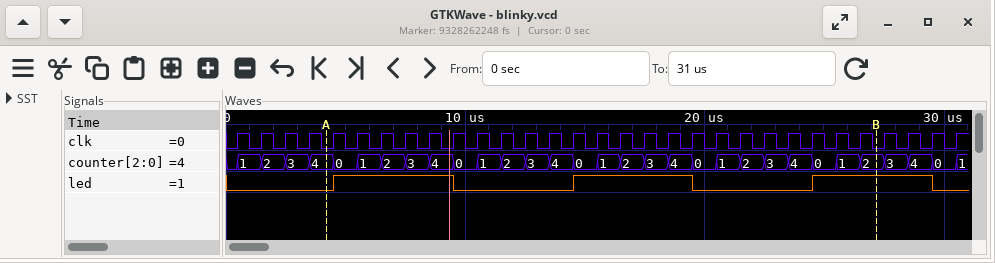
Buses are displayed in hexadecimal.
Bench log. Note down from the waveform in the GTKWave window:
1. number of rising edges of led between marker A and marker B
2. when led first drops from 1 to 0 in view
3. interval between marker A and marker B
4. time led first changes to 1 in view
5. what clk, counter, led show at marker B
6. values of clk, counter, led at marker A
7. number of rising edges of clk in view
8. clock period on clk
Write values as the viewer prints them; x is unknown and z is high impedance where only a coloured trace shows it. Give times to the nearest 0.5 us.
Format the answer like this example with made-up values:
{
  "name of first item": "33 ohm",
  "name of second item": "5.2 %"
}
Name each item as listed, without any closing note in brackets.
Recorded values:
{
  "number of rising edges of led between marker A and marker B": "3",
  "when led first drops from 1 to 0 in view": "9.5 us",
  "interval between marker A and marker B": "23 us",
  "time led first changes to 1 in view": "4.5 us",
  "what clk, counter, led show at marker B": "clk=0, counter=2, led=1",
  "values of clk, counter, led at marker A": "clk=0, counter=4, led=0",
  "number of rising edges of clk in view": "31",
  "clock period on clk": "1 us"
}
